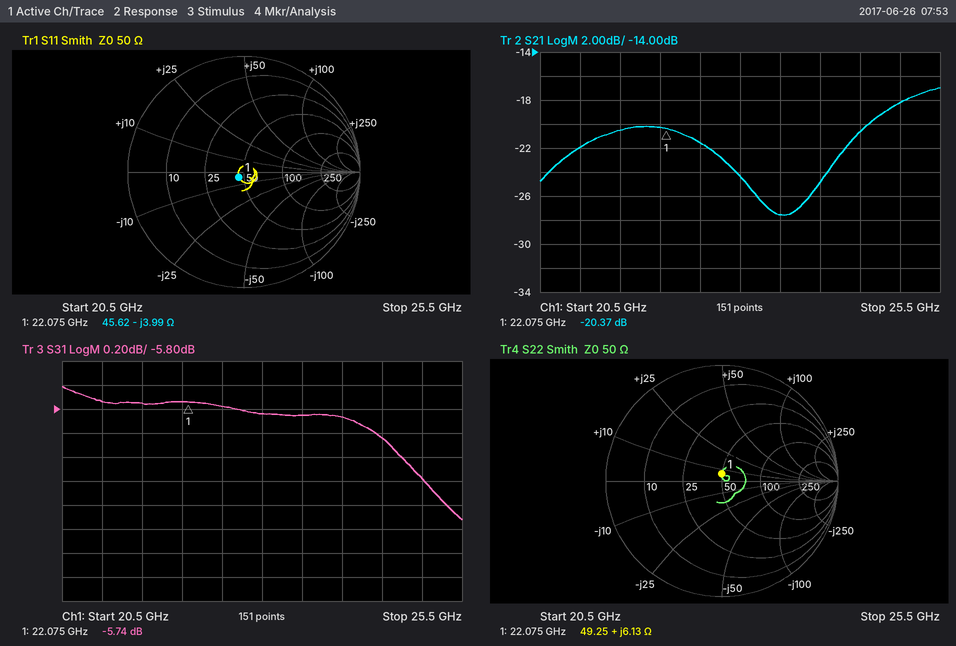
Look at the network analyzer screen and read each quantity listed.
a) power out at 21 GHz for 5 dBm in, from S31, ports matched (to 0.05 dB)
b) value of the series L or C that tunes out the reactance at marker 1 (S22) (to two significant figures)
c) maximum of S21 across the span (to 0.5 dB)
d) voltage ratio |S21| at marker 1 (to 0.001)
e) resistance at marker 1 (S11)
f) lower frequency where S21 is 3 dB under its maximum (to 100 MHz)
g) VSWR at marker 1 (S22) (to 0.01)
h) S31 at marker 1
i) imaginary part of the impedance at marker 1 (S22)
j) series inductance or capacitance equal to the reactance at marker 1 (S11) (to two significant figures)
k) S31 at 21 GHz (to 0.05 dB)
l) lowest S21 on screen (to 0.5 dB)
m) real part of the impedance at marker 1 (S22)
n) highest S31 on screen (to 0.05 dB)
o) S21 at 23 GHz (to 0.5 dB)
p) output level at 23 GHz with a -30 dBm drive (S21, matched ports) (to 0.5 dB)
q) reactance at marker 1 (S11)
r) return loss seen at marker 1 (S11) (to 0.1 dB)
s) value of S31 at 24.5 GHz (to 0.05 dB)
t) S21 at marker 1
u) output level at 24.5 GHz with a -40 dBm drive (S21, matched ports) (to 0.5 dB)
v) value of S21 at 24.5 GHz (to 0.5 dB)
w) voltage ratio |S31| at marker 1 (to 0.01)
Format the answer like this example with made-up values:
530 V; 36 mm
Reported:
-0.75 dBm; 1.2 pF; -17.0 dB; 0.096; 45.62 Ω; 24.6 GHz; 1.13; -5.74 dB; +6.13 Ω; 1.8 pF; -5.75 dB; -27.5 dB; 49.25 Ω; -5.60 dB; -24.5 dB; -54.5 dBm; -3.99 Ω; 24.2 dB; -6.05 dB; -20.37 dB; -60.5 dBm; -20.5 dB; 0.52
